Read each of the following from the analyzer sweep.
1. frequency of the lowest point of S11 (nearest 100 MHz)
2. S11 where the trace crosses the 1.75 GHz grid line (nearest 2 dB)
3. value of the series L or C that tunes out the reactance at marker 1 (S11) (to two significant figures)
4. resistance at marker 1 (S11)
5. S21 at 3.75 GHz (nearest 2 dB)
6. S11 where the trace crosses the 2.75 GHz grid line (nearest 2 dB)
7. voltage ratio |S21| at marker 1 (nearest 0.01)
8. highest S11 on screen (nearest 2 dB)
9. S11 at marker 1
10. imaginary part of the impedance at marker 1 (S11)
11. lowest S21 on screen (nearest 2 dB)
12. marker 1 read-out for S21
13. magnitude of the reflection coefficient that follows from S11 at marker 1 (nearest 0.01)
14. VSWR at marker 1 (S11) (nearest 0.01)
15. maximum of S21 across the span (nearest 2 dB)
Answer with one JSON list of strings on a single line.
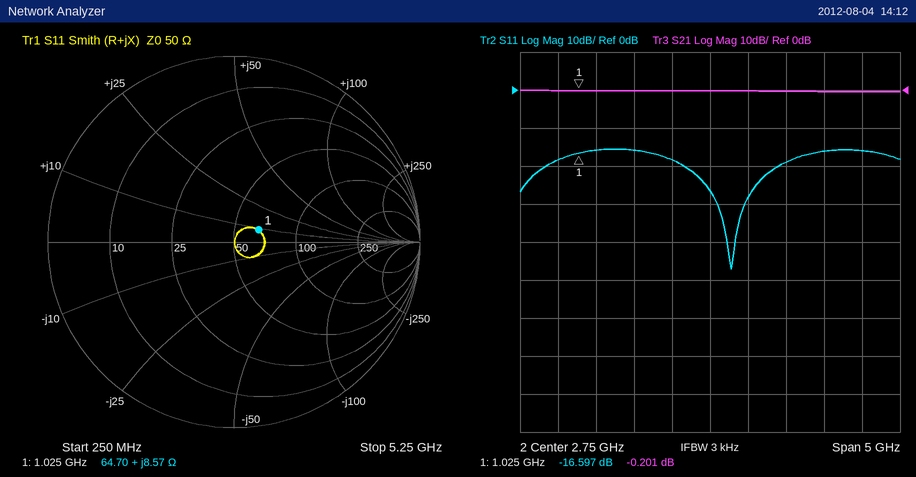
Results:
["3.0 GHz", "-16 dB", "18 pF", "64.70 Ω", "0 dB", "-26 dB", "0.98", "-16 dB", "-16.597 dB", "+8.57 Ω", "0 dB", "-0.201 dB", "0.15", "1.35", "0 dB"]
